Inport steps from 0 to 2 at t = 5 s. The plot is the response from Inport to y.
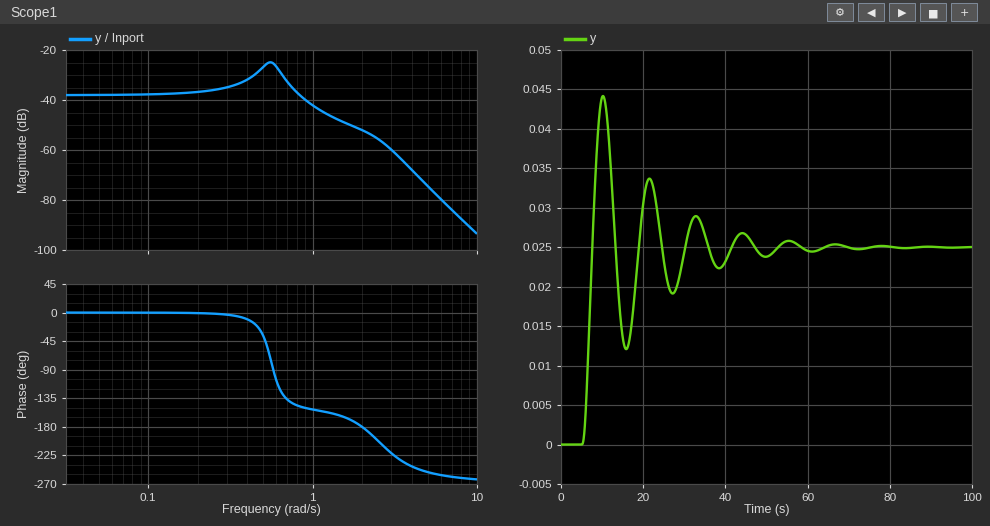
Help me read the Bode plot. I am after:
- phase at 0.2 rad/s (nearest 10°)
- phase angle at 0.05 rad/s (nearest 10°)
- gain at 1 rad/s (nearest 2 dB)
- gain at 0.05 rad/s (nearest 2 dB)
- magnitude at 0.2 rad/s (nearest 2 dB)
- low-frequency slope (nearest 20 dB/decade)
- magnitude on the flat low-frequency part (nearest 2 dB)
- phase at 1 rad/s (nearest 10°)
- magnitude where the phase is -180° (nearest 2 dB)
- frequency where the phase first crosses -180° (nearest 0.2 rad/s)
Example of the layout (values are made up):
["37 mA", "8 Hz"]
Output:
["0°", "0°", "-42 dB", "-38 dB", "-36 dB", "0 dB/decade", "-38 dB", "-150°", "-52 dB", "2.0 rad/s"]
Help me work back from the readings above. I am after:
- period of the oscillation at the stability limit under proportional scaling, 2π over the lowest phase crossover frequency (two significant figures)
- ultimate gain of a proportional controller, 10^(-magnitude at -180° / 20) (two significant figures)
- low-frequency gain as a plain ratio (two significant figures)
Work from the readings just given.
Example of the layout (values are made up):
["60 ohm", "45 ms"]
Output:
["3.1 s", "400", "0.013"]
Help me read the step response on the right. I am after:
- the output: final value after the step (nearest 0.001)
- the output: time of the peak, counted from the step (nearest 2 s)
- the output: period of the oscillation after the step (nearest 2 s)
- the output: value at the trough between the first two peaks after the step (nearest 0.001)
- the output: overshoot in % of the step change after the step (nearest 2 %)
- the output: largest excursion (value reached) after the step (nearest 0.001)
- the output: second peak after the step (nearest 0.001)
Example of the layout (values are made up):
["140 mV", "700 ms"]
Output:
["0.025", "6 s", "12 s", "0.012", "76 %", "0.044", "0.034"]
